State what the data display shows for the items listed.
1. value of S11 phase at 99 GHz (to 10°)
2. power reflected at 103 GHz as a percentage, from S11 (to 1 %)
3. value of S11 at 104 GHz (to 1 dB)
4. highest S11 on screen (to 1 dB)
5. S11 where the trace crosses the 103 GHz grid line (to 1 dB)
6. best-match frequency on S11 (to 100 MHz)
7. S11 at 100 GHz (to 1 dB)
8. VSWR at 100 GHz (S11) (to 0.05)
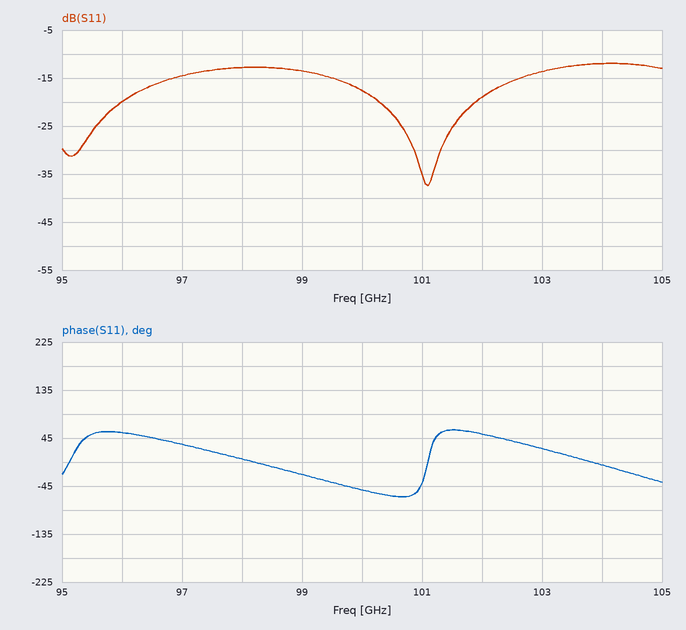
-20°
4 %
-12 dB
-12 dB
-14 dB
101.1 GHz
-18 dB
1.30
